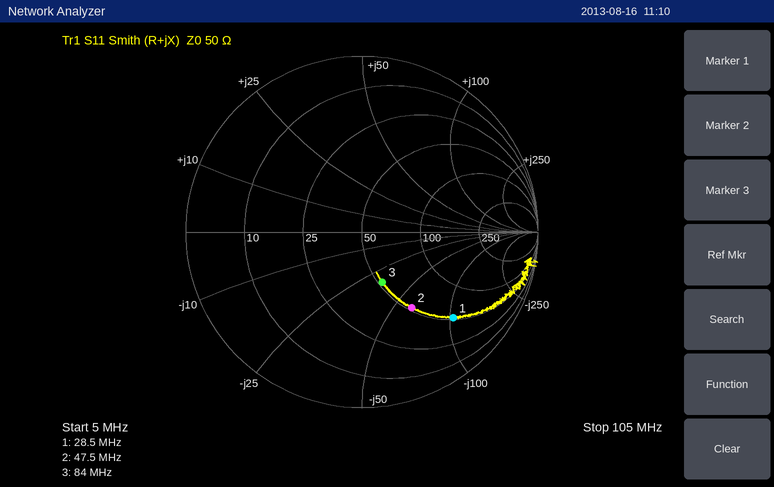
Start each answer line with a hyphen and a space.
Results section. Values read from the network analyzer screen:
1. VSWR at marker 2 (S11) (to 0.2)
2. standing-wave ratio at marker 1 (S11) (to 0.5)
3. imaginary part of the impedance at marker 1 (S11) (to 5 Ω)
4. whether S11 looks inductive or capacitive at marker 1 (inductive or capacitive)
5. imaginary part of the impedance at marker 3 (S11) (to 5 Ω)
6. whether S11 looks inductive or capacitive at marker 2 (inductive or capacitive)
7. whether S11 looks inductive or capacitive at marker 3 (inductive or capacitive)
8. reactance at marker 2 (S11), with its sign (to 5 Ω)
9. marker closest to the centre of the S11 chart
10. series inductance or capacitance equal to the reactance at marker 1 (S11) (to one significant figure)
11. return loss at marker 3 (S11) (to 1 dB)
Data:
- 3.2
- 6.0
- -105 Ω
- capacitive
- -35 Ω
- capacitive
- capacitive
- -60 Ω
- marker 3
- 50 pF
- 10 dB
